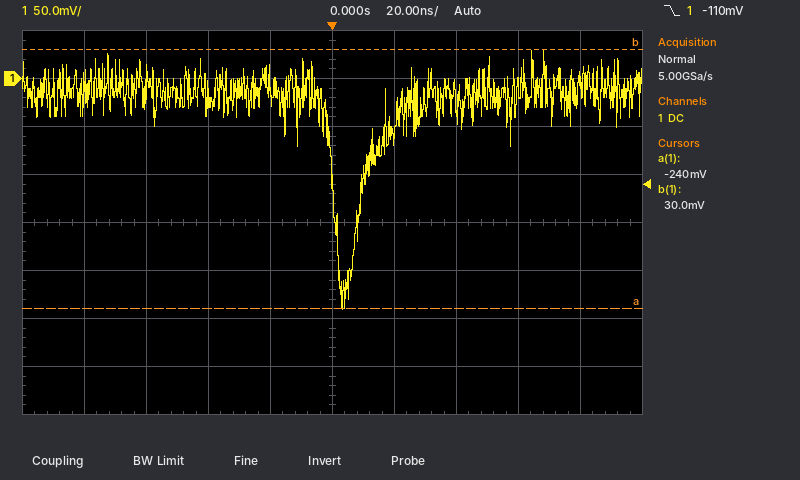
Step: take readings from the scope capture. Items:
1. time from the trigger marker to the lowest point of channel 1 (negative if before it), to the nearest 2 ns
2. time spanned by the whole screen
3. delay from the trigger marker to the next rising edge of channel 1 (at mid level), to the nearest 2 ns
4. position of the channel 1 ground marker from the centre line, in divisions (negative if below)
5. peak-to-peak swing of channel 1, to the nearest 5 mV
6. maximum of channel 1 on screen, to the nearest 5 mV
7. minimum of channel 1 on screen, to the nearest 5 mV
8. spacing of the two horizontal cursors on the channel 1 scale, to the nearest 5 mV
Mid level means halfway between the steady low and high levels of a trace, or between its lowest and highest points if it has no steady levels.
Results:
+4 ns
200 ns
10 ns
+3.0 div
270 mV
30 mV
-240 mV
270 mV
